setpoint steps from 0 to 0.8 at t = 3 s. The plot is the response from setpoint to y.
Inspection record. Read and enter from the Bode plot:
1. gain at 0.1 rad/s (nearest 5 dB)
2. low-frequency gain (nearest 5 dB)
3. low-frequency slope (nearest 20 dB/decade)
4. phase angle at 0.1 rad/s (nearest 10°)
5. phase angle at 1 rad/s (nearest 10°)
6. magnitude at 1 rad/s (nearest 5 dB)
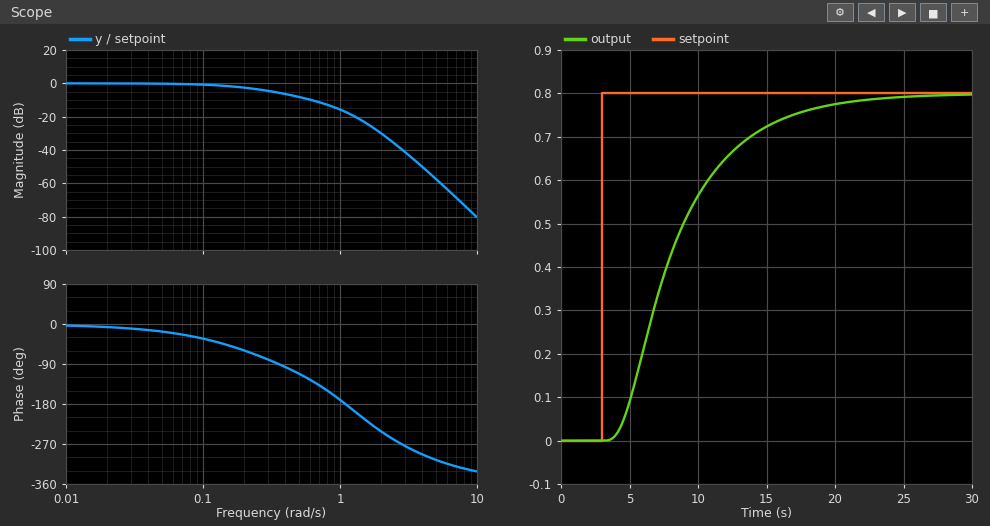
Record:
0 dB
0 dB
0 dB/decade
-30°
-170°
-15 dB
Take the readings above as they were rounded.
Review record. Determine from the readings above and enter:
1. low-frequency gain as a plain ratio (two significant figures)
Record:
1.0
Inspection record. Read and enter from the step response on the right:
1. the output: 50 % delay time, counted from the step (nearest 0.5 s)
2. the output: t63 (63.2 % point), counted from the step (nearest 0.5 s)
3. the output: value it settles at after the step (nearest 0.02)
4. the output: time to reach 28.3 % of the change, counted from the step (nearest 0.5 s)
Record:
4.5 s
6.0 s
0.80
3.0 s
